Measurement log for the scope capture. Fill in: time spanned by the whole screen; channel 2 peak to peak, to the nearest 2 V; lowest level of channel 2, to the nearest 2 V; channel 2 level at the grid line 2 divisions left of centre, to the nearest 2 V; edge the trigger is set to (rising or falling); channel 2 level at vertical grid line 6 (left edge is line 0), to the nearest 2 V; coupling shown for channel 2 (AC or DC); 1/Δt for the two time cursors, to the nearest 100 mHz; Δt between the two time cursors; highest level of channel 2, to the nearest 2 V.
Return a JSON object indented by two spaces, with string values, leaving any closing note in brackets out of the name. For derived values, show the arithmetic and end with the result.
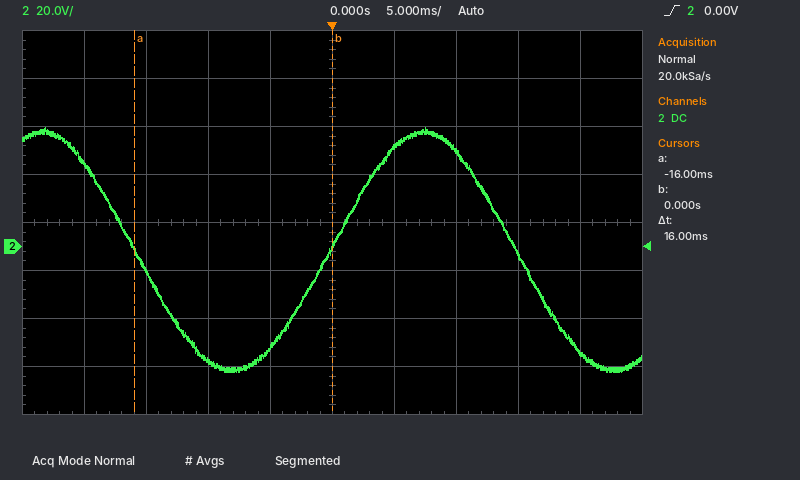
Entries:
{
  "time spanned by the whole screen": "50 ms",
  "channel 2 peak to peak, to the nearest 2 V": "50 V − (-52 V) = 102 V",
  "lowest level of channel 2, to the nearest 2 V": "-52 V",
  "channel 2 level at the grid line 2 divisions left of centre, to the nearest 2 V": "-48 V",
  "edge the trigger is set to": "rising",
  "channel 2 level at vertical grid line 6 (left edge is line 0), to the nearest 2 V": "42 V",
  "coupling shown for channel 2": "DC",
  "1/Δt for the two time cursors, to the nearest 100 mHz": "1 / 16 ms ≈ 62.5 Hz",
  "Δt between the two time cursors": "16 ms",
  "highest level of channel 2, to the nearest 2 V": "50 V"
}
